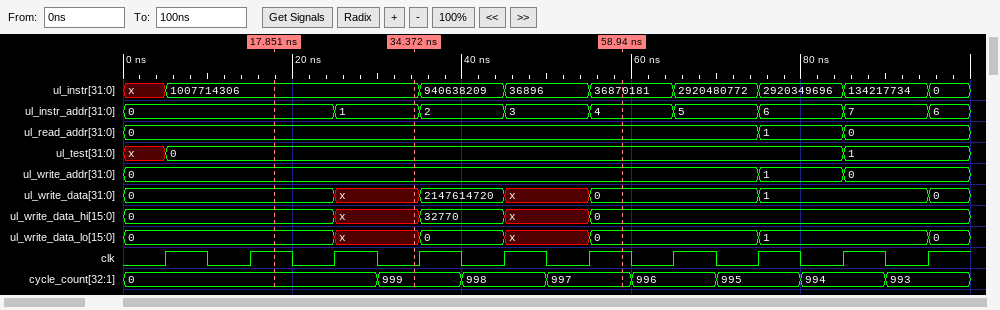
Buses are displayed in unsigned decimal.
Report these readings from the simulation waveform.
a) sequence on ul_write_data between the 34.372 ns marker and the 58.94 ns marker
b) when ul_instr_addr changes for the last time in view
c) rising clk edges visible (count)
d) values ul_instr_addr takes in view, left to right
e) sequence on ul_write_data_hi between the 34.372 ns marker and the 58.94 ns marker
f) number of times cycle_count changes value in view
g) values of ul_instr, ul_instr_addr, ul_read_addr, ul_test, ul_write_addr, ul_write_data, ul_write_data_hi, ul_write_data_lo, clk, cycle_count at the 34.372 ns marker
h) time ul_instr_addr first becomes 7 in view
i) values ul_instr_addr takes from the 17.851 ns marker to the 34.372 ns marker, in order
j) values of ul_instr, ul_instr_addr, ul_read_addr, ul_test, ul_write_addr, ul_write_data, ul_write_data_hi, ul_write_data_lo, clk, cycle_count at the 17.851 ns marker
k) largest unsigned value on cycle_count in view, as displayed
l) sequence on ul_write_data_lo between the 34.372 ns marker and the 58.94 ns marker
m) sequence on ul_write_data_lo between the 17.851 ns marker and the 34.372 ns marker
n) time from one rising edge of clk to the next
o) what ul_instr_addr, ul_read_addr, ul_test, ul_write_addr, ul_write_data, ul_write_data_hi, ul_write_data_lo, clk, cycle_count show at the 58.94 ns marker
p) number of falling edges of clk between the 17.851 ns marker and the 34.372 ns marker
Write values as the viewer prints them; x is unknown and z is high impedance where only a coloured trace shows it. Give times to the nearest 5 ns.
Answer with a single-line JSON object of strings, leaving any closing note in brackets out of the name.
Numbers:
{"sequence on ul_write_data between the 34.372 ns marker and the 58.94 ns marker": "x, 2147614720, x, 0", "when ul_instr_addr changes for the last time in view": "95 ns", "rising clk edges visible": "10", "values ul_instr_addr takes in view, left to right": "0, 1, 2, 3, 4, 5, 6, 7, 6", "sequence on ul_write_data_hi between the 34.372 ns marker and the 58.94 ns marker": "x, 32770, x, 0", "number of times cycle_count changes value in view": "7", "values of ul_instr, ul_instr_addr, ul_read_addr, ul_test, ul_write_addr, ul_write_data, ul_write_data_hi, ul_write_data_lo, clk, cycle_count at the 34.372 ns marker": "ul_instr=1007714306, ul_instr_addr=1, ul_read_addr=0, ul_test=0, ul_write_addr=0, ul_write_data=x, ul_write_data_hi=x, ul_write_data_lo=x, clk=0, cycle_count=999", "time ul_instr_addr first becomes 7 in view": "85 ns", "values ul_instr_addr takes from the 17.851 ns marker to the 34.372 ns marker, in order": "0, 1", "values of ul_instr, ul_instr_addr, ul_read_addr, ul_test, ul_write_addr, ul_write_data, ul_write_data_hi, ul_write_data_lo, clk, cycle_count at the 17.851 ns marker": "ul_instr=1007714306, ul_instr_addr=0, ul_read_addr=0, ul_test=0, ul_write_addr=0, ul_write_data=0, ul_write_data_hi=0, ul_write_data_lo=0, clk=1, cycle_count=0", "largest unsigned value on cycle_count in view, as displayed": "999", "sequence on ul_write_data_lo between the 34.372 ns marker and the 58.94 ns marker": "x, 0, x, 0", "sequence on ul_write_data_lo between the 17.851 ns marker and the 34.372 ns marker": "0, x", "time from one rising edge of clk to the next": "10 ns", "what ul_instr_addr, ul_read_addr, ul_test, ul_write_addr, ul_write_data, ul_write_data_hi, ul_write_data_lo, clk, cycle_count show at the 58.94 ns marker": "ul_instr_addr=4, ul_read_addr=0, ul_test=0, ul_write_addr=0, ul_write_data=0, ul_write_data_hi=0, ul_write_data_lo=0, clk=1, cycle_count=997", "number of falling edges of clk between the 17.851 ns marker and the 34.372 ns marker": "2"}
